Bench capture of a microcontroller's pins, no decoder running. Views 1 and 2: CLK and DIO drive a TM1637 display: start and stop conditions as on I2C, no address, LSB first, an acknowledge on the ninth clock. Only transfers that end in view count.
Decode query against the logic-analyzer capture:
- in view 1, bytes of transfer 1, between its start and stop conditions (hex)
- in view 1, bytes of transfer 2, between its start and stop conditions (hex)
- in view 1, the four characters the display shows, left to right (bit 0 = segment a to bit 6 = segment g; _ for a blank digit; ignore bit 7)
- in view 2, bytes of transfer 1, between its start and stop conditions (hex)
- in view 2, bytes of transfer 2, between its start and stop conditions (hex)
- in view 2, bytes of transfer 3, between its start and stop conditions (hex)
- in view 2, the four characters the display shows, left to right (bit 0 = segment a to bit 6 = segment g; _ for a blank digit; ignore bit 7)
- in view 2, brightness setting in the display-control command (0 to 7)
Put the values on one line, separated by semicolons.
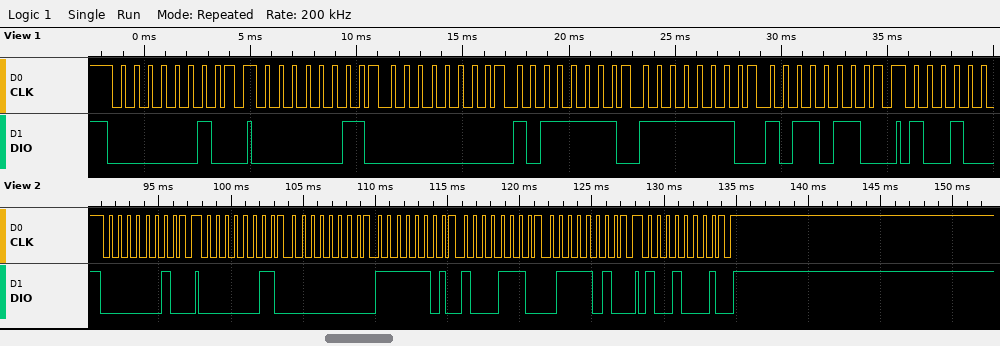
40; C0 00 FD 7F 6D; _685; 40; C0 00 BF 71 5E; 89; _0Fd; 1
